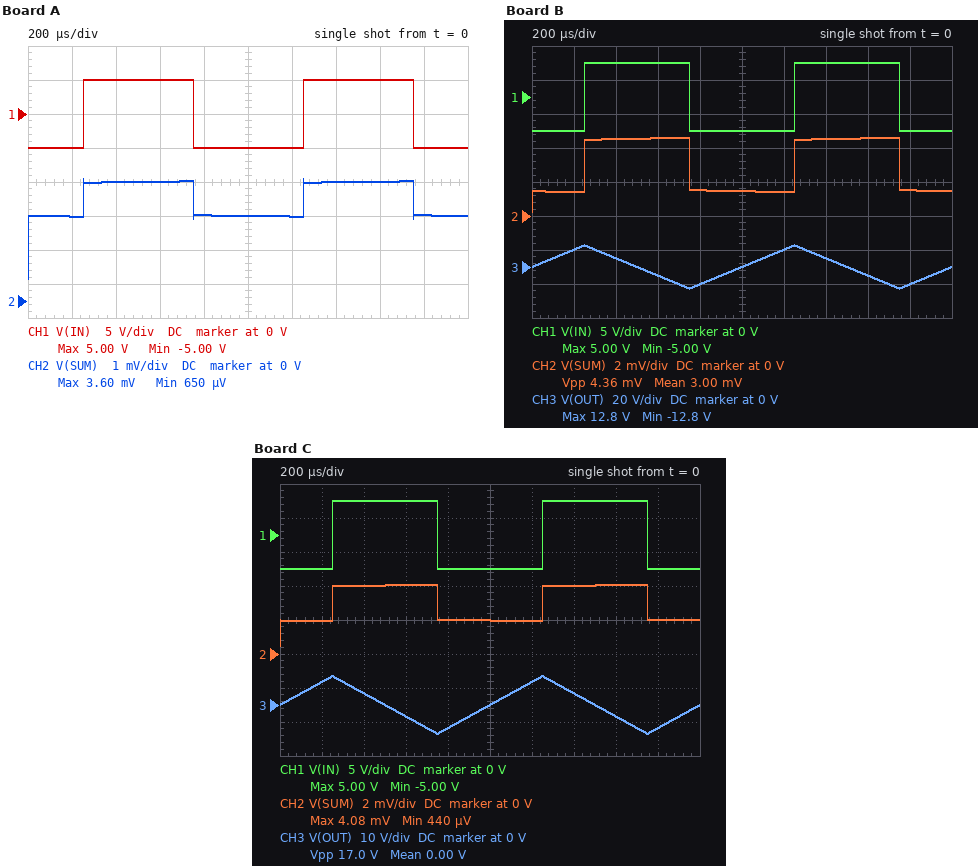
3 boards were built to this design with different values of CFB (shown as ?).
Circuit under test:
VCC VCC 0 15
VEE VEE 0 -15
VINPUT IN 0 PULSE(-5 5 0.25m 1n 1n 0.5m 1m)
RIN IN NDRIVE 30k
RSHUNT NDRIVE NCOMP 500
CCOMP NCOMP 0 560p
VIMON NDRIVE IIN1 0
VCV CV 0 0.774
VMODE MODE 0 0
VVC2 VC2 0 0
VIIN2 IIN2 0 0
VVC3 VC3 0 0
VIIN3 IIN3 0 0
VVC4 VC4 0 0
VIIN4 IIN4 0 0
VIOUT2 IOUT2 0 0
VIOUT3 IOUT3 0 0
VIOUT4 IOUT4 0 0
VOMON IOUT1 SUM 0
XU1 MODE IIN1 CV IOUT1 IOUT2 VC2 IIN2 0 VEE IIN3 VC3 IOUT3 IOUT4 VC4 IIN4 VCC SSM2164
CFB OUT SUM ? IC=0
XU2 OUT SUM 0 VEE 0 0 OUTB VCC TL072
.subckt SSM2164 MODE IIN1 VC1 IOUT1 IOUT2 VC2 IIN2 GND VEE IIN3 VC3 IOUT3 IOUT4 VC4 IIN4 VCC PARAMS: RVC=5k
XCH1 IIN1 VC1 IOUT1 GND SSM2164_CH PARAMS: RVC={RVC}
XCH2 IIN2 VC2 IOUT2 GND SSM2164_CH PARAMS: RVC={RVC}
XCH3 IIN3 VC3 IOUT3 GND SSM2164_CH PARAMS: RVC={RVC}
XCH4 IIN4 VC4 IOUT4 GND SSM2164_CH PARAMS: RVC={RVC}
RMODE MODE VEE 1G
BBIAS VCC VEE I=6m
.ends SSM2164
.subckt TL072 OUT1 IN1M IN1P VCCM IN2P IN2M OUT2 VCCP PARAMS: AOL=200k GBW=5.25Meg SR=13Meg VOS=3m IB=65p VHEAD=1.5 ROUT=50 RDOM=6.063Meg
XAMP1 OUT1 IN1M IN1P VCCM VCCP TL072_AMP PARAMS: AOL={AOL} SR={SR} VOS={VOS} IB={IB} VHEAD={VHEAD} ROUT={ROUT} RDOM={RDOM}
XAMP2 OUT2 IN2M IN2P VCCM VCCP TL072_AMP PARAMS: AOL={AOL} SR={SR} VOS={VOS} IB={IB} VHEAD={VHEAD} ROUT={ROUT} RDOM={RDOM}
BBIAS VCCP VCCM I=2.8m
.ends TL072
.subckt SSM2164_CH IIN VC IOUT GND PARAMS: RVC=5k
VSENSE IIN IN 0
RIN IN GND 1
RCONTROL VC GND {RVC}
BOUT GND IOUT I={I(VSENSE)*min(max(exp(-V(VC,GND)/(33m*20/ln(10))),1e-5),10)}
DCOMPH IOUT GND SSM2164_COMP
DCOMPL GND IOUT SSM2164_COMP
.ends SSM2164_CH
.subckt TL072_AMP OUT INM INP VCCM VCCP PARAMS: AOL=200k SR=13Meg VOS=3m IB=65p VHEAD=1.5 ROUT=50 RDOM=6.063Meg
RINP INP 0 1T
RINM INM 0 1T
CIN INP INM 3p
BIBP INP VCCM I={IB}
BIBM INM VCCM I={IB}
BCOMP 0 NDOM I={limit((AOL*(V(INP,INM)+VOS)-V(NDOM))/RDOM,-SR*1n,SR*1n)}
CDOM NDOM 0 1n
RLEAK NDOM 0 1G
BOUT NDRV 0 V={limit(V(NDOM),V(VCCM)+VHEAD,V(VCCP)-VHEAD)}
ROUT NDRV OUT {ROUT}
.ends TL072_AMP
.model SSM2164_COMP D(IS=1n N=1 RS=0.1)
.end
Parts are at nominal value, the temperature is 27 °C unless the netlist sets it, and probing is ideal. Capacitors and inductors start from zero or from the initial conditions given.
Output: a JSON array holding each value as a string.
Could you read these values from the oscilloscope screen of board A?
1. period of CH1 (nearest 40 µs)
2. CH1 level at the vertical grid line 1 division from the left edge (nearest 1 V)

["1.00 ms", "-5 V"]
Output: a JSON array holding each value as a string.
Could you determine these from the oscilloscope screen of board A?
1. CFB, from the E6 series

["680 pF"]
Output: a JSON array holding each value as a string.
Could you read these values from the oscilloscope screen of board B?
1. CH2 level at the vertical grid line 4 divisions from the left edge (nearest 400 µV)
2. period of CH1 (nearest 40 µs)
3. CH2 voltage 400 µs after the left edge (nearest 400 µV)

["1.6 mV", "1.00 ms", "4.4 mV"]
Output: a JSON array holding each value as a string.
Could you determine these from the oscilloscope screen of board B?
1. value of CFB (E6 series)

["220 pF"]
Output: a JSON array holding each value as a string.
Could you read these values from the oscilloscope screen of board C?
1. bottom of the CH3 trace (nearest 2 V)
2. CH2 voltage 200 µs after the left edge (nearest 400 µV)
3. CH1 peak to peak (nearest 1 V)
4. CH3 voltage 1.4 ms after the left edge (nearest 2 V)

["-8 V", "2.0 mV", "10 V", "4 V"]
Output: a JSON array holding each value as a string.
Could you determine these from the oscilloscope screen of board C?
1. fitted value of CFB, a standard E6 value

["330 pF"]
